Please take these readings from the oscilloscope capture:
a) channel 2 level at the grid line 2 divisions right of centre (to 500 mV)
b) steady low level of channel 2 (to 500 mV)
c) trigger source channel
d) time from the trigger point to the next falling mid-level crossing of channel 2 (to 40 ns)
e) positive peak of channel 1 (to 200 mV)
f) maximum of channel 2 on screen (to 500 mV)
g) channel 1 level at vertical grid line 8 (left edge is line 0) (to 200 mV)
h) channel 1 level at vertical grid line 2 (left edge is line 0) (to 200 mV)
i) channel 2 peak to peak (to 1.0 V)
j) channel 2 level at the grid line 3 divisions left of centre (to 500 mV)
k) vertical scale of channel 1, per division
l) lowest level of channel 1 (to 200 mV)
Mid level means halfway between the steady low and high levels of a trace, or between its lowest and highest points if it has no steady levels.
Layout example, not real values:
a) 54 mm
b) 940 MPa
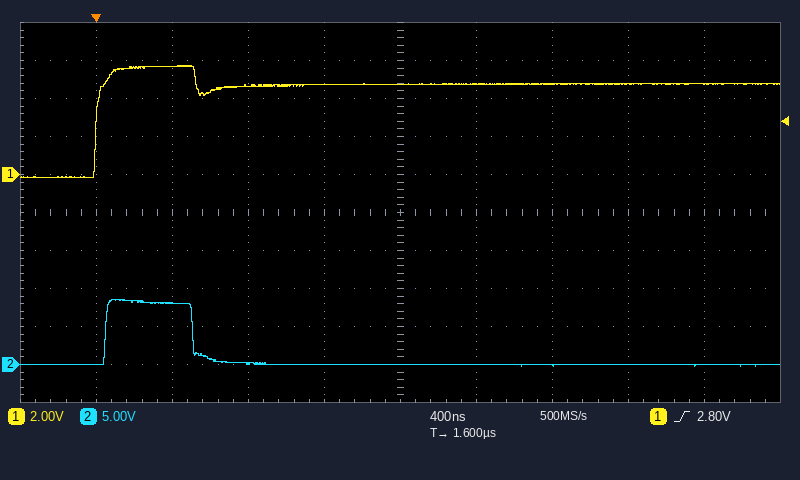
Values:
a) 0.0 V
b) 0.0 V
c) channel 1
d) 520 ns
e) 5.8 V
f) 8.5 V
g) 4.8 V
h) 5.6 V
i) 9.0 V
j) 8.0 V
k) 2 V
l) -200 mV
